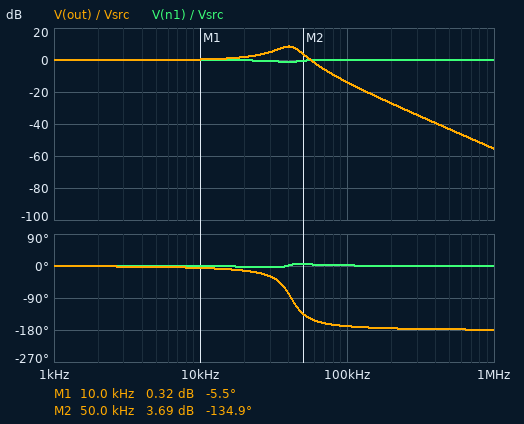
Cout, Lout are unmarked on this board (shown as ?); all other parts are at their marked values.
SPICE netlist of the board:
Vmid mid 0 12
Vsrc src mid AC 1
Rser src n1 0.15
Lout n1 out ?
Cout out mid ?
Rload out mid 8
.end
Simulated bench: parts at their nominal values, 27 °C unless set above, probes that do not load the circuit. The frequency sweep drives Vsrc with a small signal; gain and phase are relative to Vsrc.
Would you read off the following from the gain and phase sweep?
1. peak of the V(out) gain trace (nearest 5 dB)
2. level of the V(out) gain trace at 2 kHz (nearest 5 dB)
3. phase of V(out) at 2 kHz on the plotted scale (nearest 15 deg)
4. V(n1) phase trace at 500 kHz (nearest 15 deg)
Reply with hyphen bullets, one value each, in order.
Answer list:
- 10 dB
- 0 dB
- 0 deg
- 0 deg
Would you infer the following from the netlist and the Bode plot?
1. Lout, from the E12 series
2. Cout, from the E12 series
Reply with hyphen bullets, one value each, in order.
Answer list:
- 10 µH
- 1.5 µF
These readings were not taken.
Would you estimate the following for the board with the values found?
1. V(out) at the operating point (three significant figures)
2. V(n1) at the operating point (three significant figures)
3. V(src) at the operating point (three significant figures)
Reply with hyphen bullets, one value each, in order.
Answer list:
- 12.0 V
- 12.0 V
- 12.0 V
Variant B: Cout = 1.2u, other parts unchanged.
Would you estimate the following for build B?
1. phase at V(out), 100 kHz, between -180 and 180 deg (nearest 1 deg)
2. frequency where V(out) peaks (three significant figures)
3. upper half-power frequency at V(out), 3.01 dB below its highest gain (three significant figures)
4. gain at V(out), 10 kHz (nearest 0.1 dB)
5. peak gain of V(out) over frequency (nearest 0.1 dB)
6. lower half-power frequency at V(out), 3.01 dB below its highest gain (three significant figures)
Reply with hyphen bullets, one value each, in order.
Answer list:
- -166 deg
- 44.4 kHz
- 53.2 kHz
- 0.2 dB
- 7.8 dB
- 33.3 kHz
